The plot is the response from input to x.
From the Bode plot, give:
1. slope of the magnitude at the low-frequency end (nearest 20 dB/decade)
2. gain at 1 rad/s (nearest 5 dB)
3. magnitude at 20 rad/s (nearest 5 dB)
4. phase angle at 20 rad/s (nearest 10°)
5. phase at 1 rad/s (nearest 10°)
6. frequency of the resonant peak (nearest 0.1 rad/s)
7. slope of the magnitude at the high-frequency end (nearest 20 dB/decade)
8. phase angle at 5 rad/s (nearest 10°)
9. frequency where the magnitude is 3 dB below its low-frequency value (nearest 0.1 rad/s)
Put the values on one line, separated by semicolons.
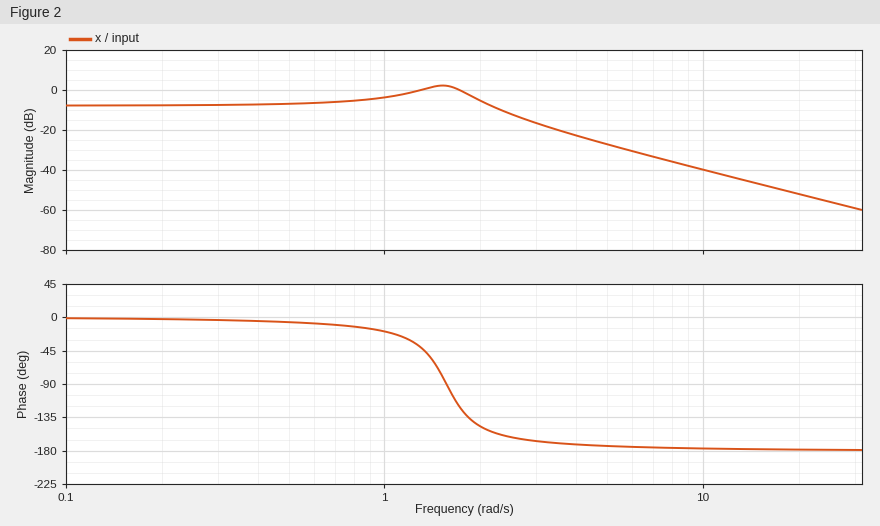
0 dB/decade; -5 dB; -50 dB; -180°; -20°; 1.5 rad/s; -40 dB/decade; -170°; 2.4 rad/s
